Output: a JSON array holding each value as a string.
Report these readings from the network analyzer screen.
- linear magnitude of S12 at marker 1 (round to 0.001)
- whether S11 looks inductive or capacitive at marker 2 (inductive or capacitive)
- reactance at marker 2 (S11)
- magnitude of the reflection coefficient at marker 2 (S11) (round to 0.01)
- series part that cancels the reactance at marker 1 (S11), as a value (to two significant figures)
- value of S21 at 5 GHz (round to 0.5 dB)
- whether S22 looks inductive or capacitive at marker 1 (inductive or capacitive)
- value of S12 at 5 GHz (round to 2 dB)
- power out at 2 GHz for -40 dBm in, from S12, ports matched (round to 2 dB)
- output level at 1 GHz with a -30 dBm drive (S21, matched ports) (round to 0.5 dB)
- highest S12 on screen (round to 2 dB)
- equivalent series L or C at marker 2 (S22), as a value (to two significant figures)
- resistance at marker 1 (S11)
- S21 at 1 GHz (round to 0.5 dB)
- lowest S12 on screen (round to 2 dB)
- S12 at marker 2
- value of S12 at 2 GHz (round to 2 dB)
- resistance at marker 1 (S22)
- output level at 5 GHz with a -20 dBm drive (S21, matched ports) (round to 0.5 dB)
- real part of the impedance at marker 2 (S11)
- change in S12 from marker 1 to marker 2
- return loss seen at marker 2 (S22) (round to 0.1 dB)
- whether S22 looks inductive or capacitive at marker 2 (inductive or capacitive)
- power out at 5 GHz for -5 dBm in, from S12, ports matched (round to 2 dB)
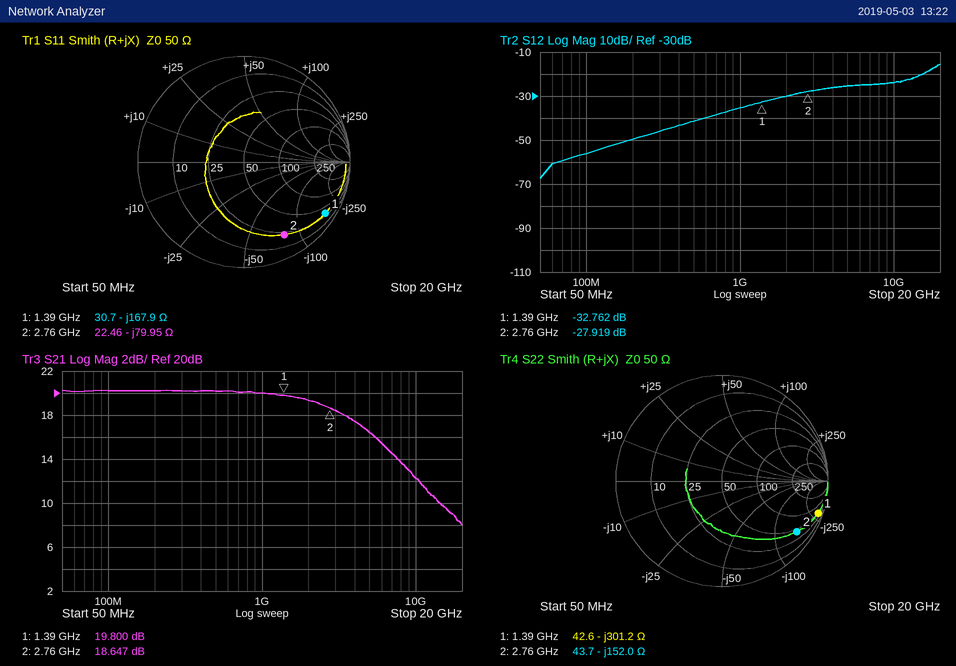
["0.023", "capacitive", "-79.95 Ω", "0.78", "19 nH", "16.5 dB", "capacitive", "-26 dB", "-70 dBm", "-10.0 dBm", "-16 dB", "380 fF", "30.7 Ω", "20.0 dB", "-68 dB", "-27.919 dB", "-30 dB", "42.6 Ω", "-3.5 dBm", "22.46 Ω", "4.843 dB", "1.4 dB", "capacitive", "-30 dBm"]
